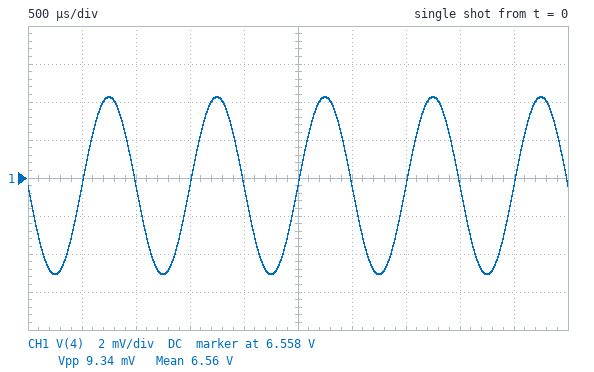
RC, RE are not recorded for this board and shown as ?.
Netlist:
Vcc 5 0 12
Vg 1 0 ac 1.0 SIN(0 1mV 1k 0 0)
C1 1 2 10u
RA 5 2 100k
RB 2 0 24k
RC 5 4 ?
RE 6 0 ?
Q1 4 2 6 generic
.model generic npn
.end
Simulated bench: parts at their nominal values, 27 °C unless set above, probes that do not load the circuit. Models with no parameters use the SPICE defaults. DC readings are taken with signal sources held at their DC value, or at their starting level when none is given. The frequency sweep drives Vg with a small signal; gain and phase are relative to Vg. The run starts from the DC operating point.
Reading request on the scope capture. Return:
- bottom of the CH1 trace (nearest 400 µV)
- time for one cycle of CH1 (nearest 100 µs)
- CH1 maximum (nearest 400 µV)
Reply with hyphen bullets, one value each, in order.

- 6.5528 V
- 1.0 ms
- 6.5624 V
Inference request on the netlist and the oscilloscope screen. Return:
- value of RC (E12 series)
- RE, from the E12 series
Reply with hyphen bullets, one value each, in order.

- 2.7 kΩ
- 560 Ω
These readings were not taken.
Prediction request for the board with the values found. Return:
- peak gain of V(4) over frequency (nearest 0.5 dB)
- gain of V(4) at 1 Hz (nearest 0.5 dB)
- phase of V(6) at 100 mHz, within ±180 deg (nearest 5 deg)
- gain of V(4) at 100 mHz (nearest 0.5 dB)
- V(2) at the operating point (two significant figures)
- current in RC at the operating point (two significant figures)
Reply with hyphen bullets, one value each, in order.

- 13.5 dB
- 10.0 dB
- 85 deg
- -7.5 dB
- 1.9 V
- 2.0 mA
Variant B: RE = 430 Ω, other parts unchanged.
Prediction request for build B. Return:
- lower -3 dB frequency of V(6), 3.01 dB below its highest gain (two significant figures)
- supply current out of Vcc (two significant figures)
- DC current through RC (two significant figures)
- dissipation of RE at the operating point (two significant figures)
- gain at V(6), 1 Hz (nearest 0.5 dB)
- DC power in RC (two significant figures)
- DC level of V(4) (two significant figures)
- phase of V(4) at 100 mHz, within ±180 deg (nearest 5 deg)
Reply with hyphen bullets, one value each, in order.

- 1.2 Hz
- 2.5 mA
- 2.4 mA
- 2.6 mW
- -4.0 dB
- 16 mW
- 5.4 V
- -95 deg
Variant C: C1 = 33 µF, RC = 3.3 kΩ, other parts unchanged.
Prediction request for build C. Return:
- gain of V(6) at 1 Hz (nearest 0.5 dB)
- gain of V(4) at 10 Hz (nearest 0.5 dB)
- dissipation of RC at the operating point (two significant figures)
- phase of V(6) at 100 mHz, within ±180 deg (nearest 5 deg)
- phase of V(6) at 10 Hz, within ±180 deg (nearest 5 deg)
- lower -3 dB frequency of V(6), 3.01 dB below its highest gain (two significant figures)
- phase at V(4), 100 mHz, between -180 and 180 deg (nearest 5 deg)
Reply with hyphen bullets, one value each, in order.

- -0.5 dB
- 15.0 dB
- 13 mW
- 75 deg
- 0 deg
- 330 mHz
- -105 deg
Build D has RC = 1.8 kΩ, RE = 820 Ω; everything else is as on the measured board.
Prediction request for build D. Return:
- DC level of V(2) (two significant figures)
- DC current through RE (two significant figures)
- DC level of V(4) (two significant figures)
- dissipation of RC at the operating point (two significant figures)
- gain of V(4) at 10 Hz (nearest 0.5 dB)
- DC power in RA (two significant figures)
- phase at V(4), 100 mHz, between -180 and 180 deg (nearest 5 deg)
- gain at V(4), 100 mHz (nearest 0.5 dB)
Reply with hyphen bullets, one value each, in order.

- 2.0 V
- 1.5 mA
- 9.3 V
- 4.1 mW
- 6.5 dB
- 990 µW
- -95 deg
- -13.5 dB
